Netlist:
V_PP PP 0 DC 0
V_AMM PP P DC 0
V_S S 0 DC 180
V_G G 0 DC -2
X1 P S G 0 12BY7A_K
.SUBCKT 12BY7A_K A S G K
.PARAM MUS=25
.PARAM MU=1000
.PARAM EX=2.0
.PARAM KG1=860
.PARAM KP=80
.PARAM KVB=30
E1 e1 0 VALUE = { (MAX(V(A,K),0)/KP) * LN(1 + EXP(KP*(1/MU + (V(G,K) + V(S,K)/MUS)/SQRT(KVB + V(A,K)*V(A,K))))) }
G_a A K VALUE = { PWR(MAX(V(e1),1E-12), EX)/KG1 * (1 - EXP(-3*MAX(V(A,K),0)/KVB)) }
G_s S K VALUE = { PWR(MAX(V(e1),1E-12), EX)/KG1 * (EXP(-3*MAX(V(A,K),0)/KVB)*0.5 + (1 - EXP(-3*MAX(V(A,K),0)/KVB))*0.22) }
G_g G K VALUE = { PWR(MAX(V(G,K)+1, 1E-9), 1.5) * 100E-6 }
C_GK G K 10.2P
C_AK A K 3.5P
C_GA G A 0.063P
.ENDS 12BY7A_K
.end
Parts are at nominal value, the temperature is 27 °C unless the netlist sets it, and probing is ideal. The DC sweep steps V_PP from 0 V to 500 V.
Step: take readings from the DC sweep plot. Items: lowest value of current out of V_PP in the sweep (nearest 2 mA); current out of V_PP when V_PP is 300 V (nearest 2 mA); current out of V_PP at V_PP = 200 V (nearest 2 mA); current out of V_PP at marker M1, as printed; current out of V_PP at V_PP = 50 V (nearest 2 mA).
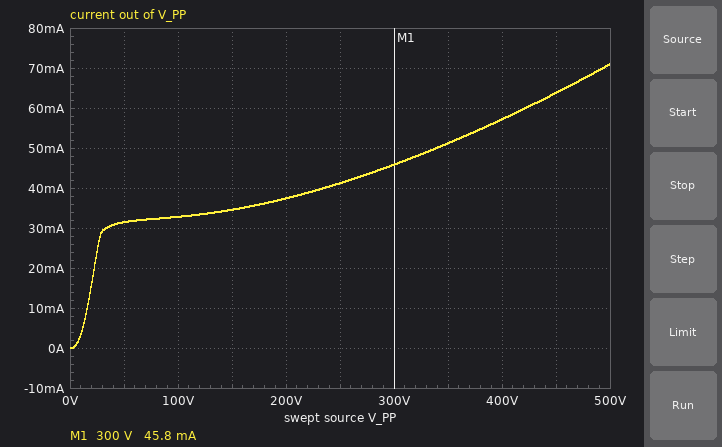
0 A
46 mA
38 mA
45.8 mA
32 mA
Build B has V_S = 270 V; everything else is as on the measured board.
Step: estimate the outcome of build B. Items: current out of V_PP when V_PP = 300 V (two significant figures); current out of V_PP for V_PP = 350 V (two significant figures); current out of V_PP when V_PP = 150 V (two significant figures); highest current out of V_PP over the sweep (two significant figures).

100 mA
110 mA
93 mA
130 mA
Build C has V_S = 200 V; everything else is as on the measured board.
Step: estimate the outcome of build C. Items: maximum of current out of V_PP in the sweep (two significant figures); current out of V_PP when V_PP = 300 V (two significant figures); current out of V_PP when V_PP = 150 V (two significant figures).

82 mA
56 mA
45 mA
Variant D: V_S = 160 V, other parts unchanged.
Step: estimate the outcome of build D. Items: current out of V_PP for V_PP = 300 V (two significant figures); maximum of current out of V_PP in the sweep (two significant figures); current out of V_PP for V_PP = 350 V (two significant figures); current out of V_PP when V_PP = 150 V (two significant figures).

37 mA
61 mA
42 mA
26 mA
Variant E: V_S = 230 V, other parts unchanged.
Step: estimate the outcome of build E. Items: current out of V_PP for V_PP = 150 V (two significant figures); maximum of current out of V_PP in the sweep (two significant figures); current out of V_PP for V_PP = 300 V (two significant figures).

63 mA
100 mA
74 mA
